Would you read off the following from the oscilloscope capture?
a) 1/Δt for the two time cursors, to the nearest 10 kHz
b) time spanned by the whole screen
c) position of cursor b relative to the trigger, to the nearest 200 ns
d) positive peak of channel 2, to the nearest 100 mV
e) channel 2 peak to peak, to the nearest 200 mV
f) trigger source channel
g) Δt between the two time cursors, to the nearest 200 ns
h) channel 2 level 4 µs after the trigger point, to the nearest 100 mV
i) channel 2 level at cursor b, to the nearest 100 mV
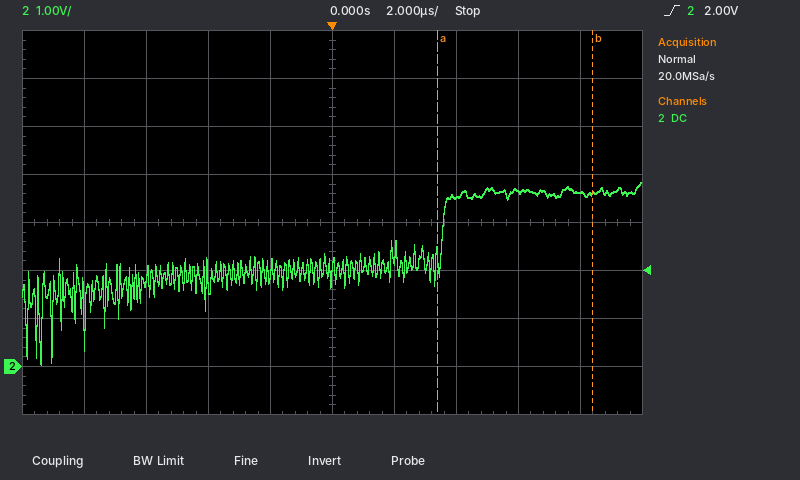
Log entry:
200 kHz
20 µs
+8.4 µs
3.8 V
3.8 V
channel 2
5.0 µs
3.5 V
3.6 V
